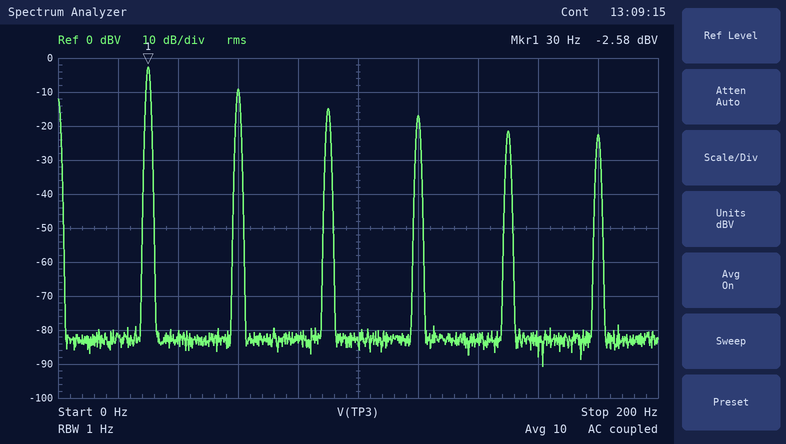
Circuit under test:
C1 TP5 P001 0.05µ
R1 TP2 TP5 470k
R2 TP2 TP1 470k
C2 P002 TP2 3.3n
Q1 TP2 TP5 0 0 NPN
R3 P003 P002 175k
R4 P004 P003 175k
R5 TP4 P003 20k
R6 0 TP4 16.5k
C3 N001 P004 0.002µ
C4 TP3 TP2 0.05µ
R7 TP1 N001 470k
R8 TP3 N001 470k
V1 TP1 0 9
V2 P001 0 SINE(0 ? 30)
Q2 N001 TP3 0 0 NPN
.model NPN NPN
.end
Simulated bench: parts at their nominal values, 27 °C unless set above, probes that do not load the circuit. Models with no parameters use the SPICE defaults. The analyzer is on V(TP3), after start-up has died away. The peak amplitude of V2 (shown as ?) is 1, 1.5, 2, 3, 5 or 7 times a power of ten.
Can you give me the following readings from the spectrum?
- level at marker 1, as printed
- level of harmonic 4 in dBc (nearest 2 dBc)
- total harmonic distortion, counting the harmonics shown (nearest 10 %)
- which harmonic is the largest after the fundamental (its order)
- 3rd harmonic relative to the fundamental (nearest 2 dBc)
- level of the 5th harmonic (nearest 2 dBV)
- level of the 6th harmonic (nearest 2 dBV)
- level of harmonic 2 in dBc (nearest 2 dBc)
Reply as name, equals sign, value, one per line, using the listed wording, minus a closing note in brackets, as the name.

level at marker 1, as printed = -2.58 dBV
level of harmonic 4 in dBc = -14 dBc
total harmonic distortion, counting the harmonics shown = 60 %
which harmonic is the largest after the fundamental = 2
3rd harmonic relative to the fundamental = -12 dBc
level of the 5th harmonic = -22 dBV
level of the 6th harmonic = -22 dBV
level of harmonic 2 in dBc = -6 dBc
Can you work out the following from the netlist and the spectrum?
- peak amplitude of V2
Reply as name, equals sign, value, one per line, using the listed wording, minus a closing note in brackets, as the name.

peak amplitude of V2 = 500 mV
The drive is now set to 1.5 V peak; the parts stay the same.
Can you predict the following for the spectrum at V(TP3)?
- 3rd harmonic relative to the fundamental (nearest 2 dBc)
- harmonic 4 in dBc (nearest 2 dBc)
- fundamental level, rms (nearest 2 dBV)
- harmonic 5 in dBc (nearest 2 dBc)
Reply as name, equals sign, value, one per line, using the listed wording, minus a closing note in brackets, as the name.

3rd harmonic relative to the fundamental = -14 dBc
harmonic 4 in dBc = -12 dBc
fundamental level, rms = 0 dBV
harmonic 5 in dBc = -16 dBc
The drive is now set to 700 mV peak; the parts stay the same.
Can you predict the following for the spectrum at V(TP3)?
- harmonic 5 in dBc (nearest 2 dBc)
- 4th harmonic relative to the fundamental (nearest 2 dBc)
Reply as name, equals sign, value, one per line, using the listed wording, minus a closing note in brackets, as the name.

harmonic 5 in dBc = -16 dBc
4th harmonic relative to the fundamental = -12 dBc
